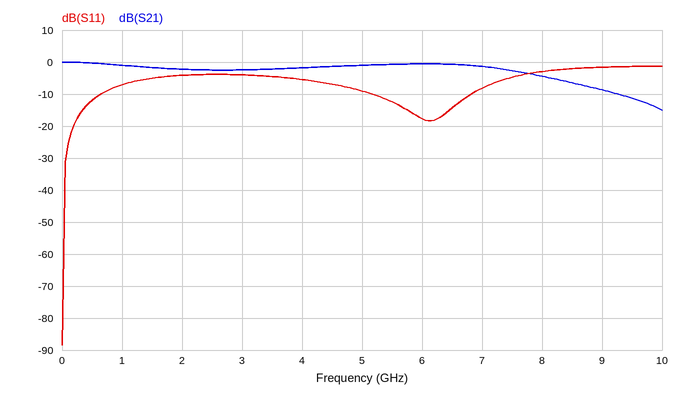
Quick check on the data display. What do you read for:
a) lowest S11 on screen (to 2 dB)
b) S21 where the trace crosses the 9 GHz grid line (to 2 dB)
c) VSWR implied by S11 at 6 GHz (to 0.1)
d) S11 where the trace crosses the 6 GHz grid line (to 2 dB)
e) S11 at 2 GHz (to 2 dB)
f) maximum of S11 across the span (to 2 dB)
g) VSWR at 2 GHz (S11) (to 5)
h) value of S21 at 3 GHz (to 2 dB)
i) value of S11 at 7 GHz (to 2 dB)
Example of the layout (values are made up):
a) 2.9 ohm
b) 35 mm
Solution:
a) -88 dB
b) -8 dB
c) 1.3
d) -18 dB
e) -4 dB
f) -2 dB
g) 5
h) -2 dB
i) -8 dB
